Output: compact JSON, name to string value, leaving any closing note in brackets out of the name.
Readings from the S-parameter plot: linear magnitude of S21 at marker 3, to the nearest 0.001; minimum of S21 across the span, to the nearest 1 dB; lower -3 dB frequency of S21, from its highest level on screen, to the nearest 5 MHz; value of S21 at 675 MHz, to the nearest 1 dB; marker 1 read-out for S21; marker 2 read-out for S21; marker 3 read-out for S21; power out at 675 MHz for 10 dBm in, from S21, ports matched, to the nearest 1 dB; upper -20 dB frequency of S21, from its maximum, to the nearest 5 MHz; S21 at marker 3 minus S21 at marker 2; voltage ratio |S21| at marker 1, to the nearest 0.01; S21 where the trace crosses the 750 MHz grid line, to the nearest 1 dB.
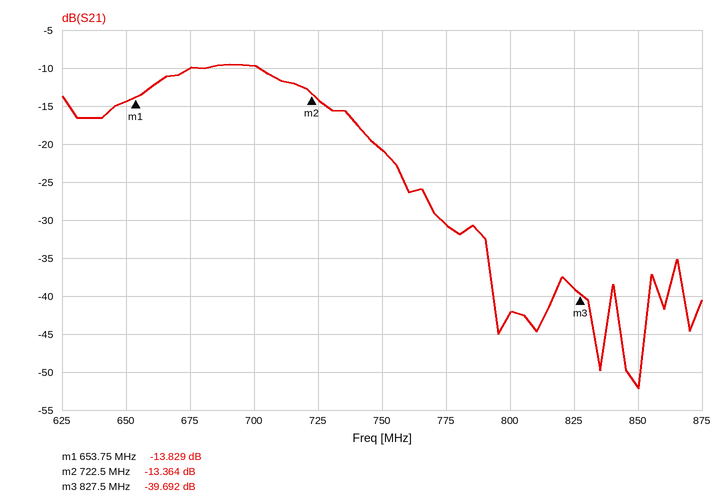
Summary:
{"linear magnitude of S21 at marker 3, to the nearest 0.001": "0.010", "minimum of S21 across the span, to the nearest 1 dB": "-52 dB", "lower -3 dB frequency of S21, from its highest level on screen, to the nearest 5 MHz": "660 MHz", "value of S21 at 675 MHz, to the nearest 1 dB": "-10 dB", "marker 1 read-out for S21": "-13.829 dB", "marker 2 read-out for S21": "-13.364 dB", "marker 3 read-out for S21": "-39.692 dB", "power out at 675 MHz for 10 dBm in, from S21, ports matched, to the nearest 1 dB": "0 dBm", "upper -20 dB frequency of S21, from its maximum, to the nearest 5 MHz": "770 MHz", "S21 at marker 3 minus S21 at marker 2": "-26.328 dB", "voltage ratio |S21| at marker 1, to the nearest 0.01": "0.20", "S21 where the trace crosses the 750 MHz grid line, to the nearest 1 dB": "-21 dB"}
